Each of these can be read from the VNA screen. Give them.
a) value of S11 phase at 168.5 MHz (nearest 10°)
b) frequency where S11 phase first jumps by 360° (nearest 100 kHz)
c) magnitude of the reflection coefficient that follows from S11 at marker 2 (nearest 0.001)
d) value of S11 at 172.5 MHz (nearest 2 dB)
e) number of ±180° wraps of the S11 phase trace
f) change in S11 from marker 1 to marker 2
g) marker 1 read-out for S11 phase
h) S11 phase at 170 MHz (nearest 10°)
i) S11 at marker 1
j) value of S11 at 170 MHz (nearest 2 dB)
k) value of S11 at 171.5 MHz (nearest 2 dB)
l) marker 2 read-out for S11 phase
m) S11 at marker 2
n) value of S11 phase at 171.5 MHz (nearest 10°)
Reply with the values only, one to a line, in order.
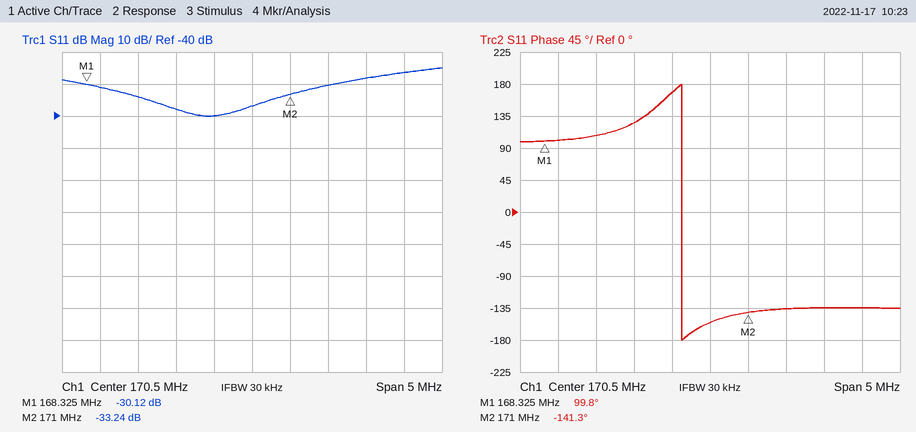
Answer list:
100°
170.1 MHz
0.022
-26 dB
1
-3.12 dB
99.8°
170°
-30.12 dB
-40 dB
-30 dB
-141.3°
-33.24 dB
-140°
